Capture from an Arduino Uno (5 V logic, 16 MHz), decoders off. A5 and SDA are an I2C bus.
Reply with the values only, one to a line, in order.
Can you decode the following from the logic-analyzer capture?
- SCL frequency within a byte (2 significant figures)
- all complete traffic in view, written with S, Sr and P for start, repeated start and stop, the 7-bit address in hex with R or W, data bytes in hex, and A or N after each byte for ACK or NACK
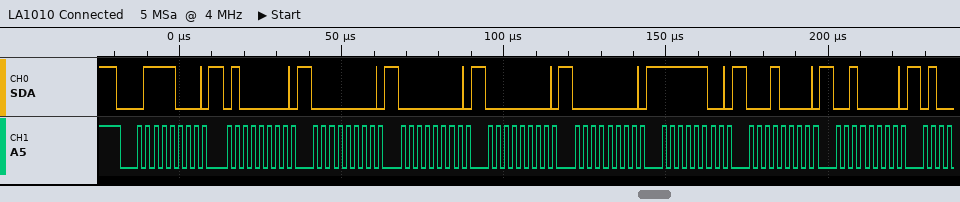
400 kHz
S 3CW A 40 A 00 A 00 A 00 A 00 A FC A 10 A 20 A
